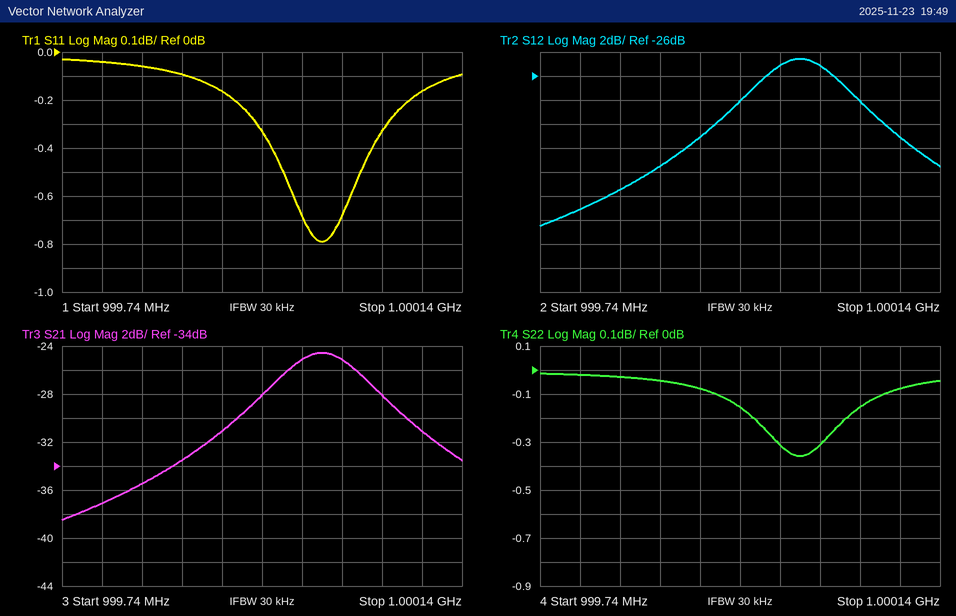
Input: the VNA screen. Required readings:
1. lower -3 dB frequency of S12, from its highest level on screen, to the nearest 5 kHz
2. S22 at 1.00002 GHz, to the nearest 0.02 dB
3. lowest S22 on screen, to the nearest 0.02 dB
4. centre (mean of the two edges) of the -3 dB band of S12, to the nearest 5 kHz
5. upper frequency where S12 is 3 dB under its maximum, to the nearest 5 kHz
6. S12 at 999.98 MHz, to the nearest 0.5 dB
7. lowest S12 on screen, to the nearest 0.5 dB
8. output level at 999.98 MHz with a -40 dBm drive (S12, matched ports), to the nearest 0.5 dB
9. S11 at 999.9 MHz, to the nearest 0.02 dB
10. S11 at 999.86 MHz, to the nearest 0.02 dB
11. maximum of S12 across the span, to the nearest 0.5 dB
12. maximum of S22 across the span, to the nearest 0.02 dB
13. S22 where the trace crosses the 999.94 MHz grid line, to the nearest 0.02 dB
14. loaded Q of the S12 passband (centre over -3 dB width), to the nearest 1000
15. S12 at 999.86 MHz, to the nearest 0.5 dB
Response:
999.945 MHz
-0.32 dB
-0.36 dB
1.000000 GHz
1.000055 GHz
-25.0 dB
-38.5 dB
-65.0 dBm
-0.16 dB
-0.10 dB
-24.5 dB
-0.02 dB
-0.16 dB
9000
-33.5 dB
